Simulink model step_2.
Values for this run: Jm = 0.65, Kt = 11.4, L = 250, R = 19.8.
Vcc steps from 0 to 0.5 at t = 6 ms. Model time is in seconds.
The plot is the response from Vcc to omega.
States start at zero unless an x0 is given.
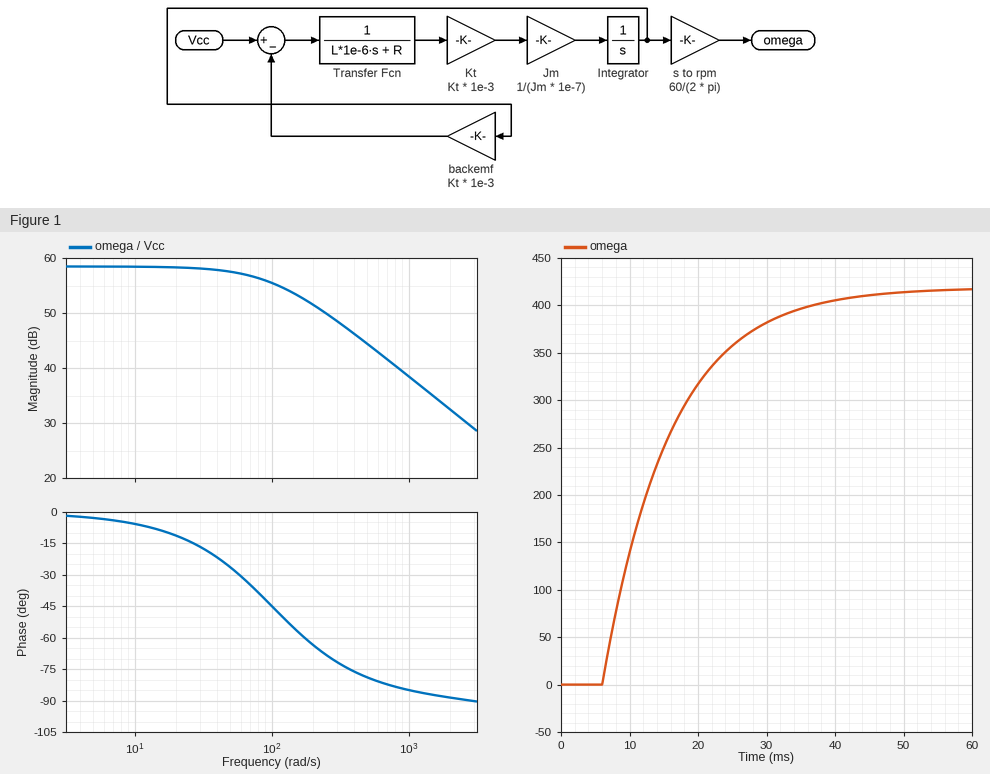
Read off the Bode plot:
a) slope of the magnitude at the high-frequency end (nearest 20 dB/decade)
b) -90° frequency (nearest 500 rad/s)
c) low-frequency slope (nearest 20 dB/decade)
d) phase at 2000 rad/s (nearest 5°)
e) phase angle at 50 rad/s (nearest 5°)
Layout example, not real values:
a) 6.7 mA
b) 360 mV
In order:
a) -20 dB/decade
b) 3000 rad/s
c) 0 dB/decade
d) -90°
e) -25°
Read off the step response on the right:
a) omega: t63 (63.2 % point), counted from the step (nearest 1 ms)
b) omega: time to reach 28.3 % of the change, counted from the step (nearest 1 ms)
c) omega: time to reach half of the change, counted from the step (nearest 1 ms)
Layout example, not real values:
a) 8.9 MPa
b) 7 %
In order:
a) 10 ms
b) 3 ms
c) 7 ms
